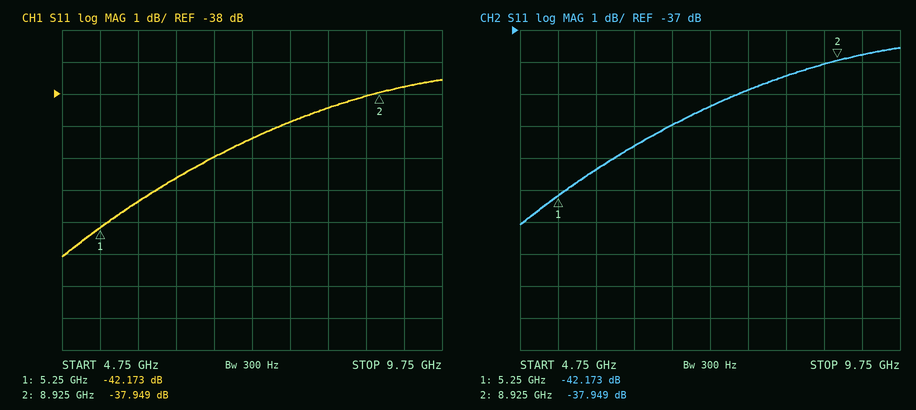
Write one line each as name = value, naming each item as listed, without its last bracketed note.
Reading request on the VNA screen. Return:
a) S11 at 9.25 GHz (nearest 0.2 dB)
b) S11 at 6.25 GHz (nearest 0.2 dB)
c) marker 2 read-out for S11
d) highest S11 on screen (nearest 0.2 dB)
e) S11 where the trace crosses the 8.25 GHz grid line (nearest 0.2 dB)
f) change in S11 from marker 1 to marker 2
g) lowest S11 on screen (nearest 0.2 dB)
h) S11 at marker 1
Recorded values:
S11 at 9.25 GHz = -37.8 dB
S11 at 6.25 GHz = -40.6 dB
marker 2 read-out for S11 = -37.949 dB
highest S11 on screen = -37.6 dB
S11 where the trace crosses the 8.25 GHz grid line = -38.4 dB
change in S11 from marker 1 to marker 2 = 4.224 dB
lowest S11 on screen = -43.0 dB
S11 at marker 1 = -42.173 dB
